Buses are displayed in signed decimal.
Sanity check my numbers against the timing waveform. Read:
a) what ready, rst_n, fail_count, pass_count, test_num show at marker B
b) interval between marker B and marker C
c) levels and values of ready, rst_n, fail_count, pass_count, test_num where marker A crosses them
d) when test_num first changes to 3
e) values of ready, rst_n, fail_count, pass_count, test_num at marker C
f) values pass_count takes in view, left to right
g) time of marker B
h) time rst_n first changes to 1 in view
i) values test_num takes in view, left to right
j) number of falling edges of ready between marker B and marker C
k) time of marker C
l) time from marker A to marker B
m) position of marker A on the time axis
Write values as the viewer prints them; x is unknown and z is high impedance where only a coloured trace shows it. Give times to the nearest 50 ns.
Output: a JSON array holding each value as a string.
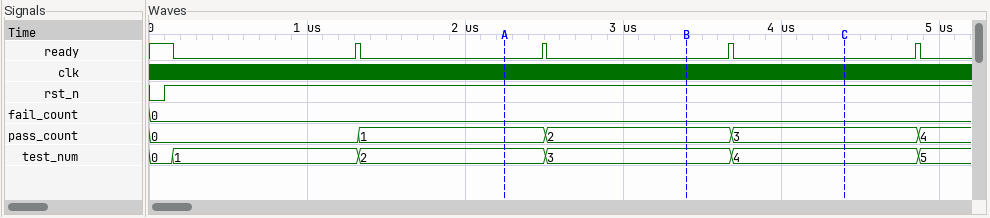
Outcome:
["ready=0, rst_n=1, fail_count=0, pass_count=2, test_num=3", "1000 ns", "ready=0, rst_n=1, fail_count=0, pass_count=1, test_num=2", "2500 ns", "ready=0, rst_n=1, fail_count=0, pass_count=3, test_num=4", "0, 1, 2, 3, 4", "3400 ns", "100 ns", "0, 1, 2, 3, 4, 5", "1", "4400 ns", "1150 ns", "2250 ns"]
